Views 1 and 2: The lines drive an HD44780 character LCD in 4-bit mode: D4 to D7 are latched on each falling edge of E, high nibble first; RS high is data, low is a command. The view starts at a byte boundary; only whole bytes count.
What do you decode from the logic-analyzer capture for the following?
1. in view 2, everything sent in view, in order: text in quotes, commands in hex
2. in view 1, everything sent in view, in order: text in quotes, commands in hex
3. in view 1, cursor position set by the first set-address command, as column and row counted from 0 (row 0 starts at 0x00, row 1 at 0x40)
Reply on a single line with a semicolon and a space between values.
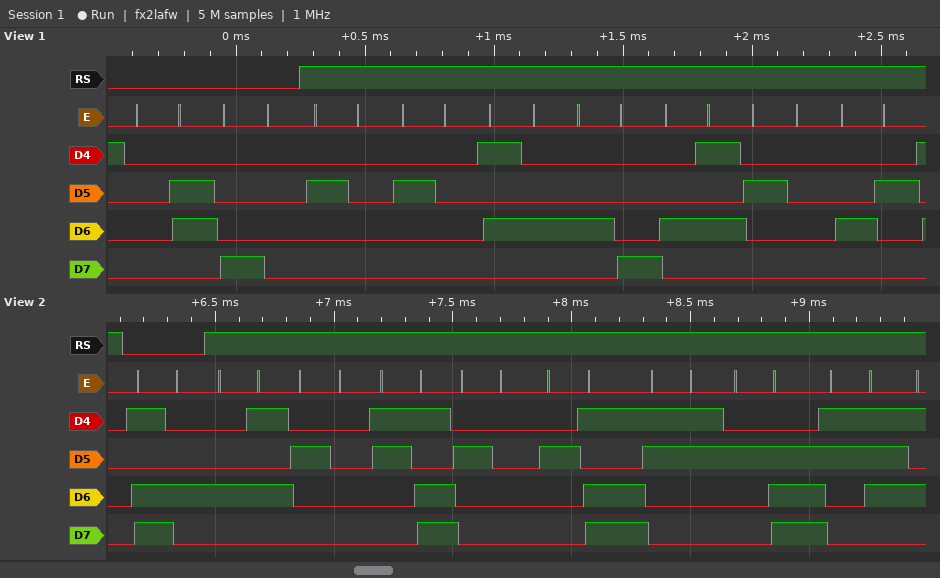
0xD4 "E = -3.7"; 0x06 0x80 "  THE B"; column 0, row 0
